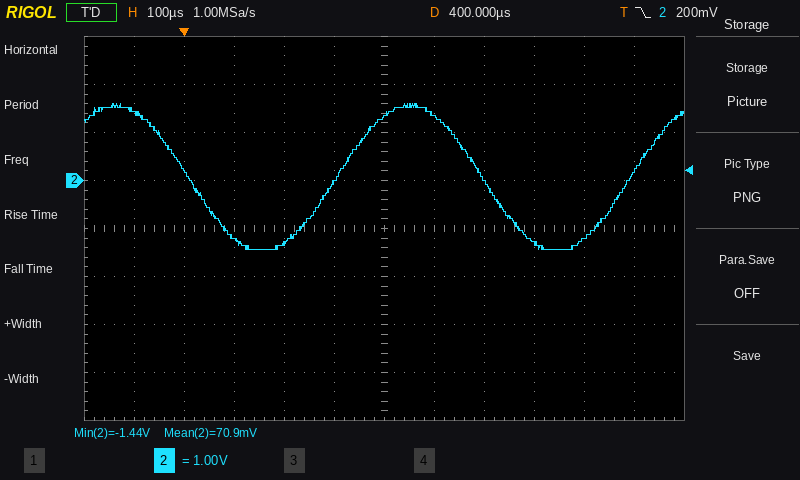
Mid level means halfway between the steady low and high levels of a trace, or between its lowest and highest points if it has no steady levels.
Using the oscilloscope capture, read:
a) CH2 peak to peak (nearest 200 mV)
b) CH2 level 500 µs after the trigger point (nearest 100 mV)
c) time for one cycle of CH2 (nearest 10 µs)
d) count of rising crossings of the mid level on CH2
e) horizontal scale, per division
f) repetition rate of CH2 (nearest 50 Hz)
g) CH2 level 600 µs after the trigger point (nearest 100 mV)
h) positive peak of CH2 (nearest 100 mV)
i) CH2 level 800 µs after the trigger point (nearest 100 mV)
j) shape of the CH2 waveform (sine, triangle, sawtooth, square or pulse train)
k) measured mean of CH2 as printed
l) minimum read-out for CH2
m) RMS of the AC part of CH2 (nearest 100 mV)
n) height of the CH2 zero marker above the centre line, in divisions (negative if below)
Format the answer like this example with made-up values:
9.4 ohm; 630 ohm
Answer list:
3.0 V; 1.4 V; 590 µs; 2; 100 µs; 1.70 kHz; 0.0 V; 1.6 V; -1.2 V; sine; 70.9 mV; -1.44 V; 1.1 V; +1.0 div
